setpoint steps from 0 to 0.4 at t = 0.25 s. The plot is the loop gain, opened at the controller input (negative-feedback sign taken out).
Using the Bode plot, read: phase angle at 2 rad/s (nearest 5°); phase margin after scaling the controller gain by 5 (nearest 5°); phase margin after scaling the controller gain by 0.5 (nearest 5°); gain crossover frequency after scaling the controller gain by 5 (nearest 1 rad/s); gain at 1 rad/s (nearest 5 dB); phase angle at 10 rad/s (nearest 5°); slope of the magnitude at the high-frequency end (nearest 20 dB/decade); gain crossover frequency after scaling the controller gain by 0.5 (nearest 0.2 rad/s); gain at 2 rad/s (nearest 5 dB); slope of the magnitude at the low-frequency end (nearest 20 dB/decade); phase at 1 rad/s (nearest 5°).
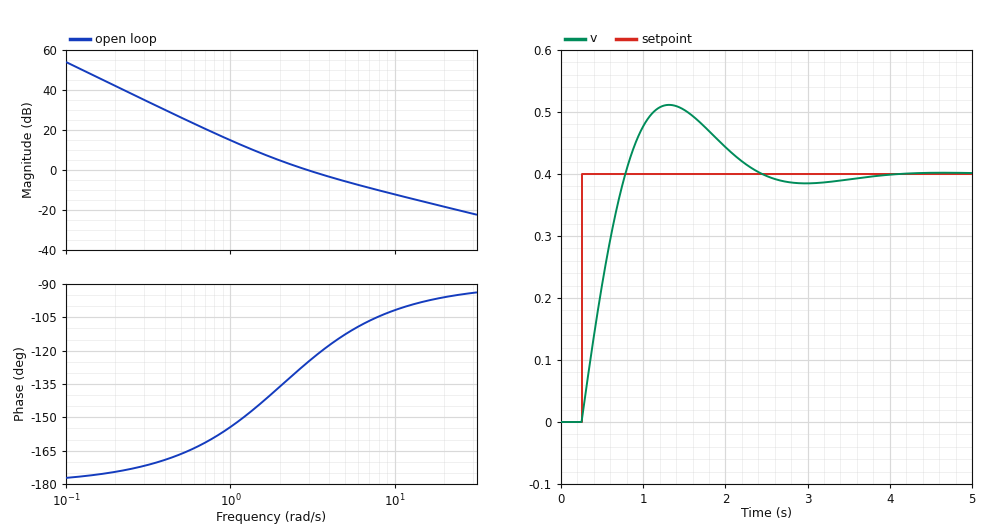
-135°
80°
40°
12 rad/s
15 dB
-100°
-20 dB/decade
1.8 rad/s
5 dB
-40 dB/decade
-155°
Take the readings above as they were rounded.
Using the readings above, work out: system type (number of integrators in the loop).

2
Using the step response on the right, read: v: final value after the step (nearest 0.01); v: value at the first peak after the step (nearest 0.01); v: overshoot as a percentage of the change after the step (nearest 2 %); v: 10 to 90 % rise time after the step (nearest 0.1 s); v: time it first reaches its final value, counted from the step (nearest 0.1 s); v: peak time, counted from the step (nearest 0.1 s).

0.40
0.51
28 %
0.4 s
0.5 s
1.1 s
